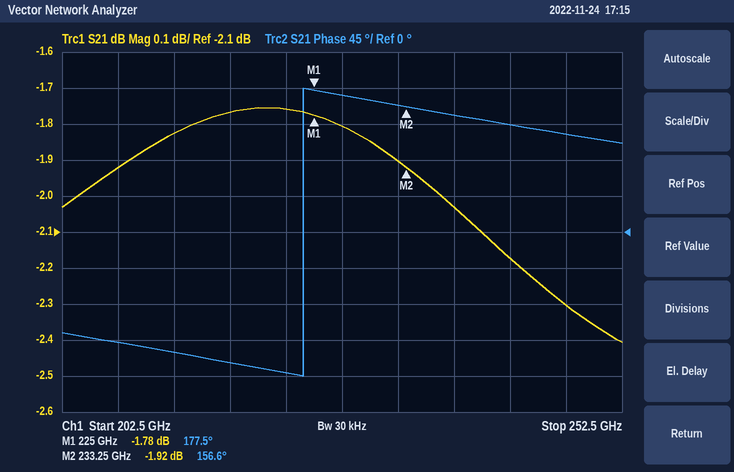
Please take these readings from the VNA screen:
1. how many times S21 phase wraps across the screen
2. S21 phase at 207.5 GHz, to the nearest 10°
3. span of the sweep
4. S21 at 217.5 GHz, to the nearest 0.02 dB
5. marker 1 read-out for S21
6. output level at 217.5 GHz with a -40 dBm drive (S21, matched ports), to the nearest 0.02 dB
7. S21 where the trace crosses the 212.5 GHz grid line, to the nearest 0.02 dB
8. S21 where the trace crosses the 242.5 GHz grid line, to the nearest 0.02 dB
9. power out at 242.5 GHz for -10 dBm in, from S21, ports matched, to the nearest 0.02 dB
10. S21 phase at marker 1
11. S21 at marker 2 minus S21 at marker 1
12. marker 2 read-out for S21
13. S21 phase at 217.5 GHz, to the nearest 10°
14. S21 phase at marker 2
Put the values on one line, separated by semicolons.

1; -140°; 50 GHz; -1.76 dB; -1.78 dB; -41.76 dBm; -1.82 dB; -2.18 dB; -12.18 dBm; 177.5°; -0.14 dB; -1.92 dB; -160°; 156.6°
